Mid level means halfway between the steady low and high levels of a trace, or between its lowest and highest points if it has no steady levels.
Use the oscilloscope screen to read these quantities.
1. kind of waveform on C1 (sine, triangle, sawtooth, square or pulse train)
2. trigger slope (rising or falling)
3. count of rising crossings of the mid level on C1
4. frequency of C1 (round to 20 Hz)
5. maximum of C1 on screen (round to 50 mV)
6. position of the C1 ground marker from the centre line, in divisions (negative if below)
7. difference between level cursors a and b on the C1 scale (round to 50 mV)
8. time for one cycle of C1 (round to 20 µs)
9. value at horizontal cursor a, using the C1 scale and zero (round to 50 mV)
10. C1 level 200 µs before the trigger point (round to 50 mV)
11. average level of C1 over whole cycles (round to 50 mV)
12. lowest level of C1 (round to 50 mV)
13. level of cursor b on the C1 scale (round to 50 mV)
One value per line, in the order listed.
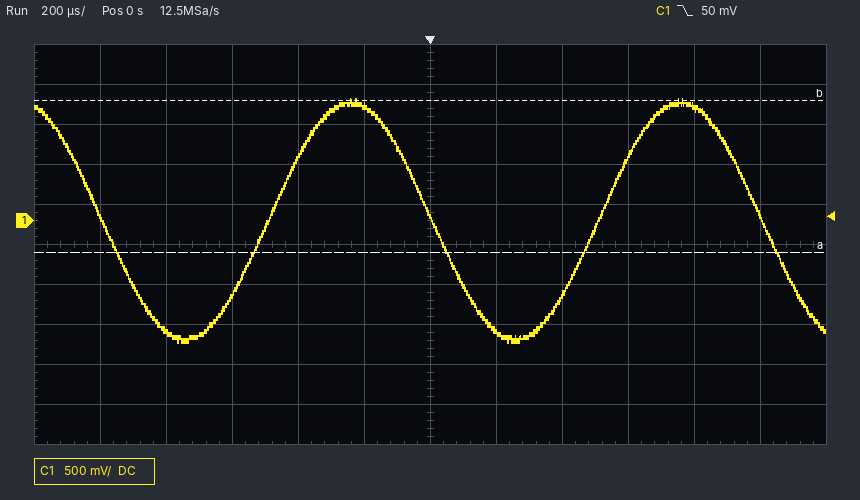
sine
falling
2
1.00 kHz
1.50 V
+0.6 div
1.90 V
1.00 ms
-400 mV
1.45 V
0 mV
-1.50 V
1.50 V
